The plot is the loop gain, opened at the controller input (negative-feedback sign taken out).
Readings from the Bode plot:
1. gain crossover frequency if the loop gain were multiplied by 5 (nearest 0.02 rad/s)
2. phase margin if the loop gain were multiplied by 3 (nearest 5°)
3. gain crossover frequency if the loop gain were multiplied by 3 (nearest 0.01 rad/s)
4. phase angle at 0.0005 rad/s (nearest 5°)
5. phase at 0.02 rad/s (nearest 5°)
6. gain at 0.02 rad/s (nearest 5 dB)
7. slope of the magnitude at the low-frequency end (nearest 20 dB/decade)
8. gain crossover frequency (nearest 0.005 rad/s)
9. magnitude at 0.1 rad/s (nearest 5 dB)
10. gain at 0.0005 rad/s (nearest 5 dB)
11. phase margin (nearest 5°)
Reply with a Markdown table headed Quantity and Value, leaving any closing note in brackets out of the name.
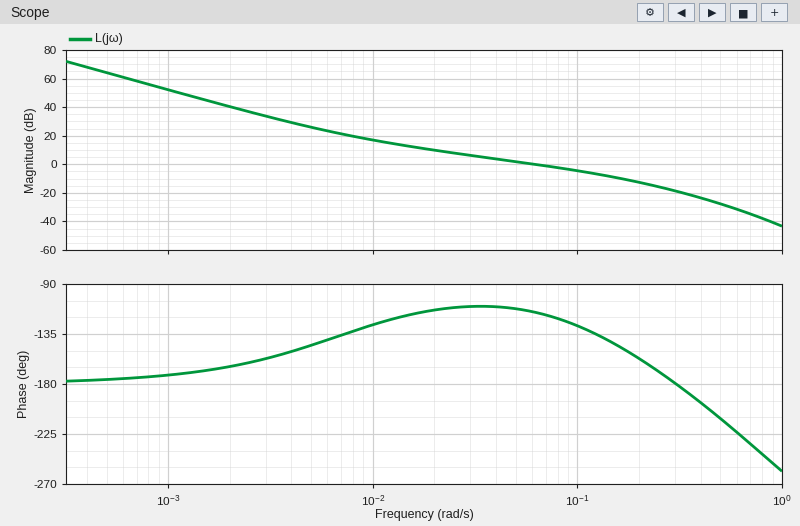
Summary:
| Quantity | Value |
|---|---|
| gain crossover frequency if the loop gain were multiplied by 5 | 0.22 rad/s |
| phase margin if the loop gain were multiplied by 3 | 35° |
| gain crossover frequency if the loop gain were multiplied by 3 | 0.16 rad/s |
| phase angle at 0.0005 rad/s | -175° |
| phase at 0.02 rad/s | -115° |
| gain at 0.02 rad/s | 10 dB |
| slope of the magnitude at the low-frequency end | -40 dB/decade |
| gain crossover frequency | 0.060 rad/s |
| magnitude at 0.1 rad/s | -5 dB |
| gain at 0.0005 rad/s | 65 dB |
| phase margin | 65° |
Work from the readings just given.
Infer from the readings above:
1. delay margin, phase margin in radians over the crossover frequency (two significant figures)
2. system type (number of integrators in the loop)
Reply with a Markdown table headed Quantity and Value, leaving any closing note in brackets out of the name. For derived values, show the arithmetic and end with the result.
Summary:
| Quantity | Value |
|---|---|
| delay margin, phase margin in radians over the crossover frequency | 65 × π / 180 / 0.06 = 19 s |
| system type | 2 |
